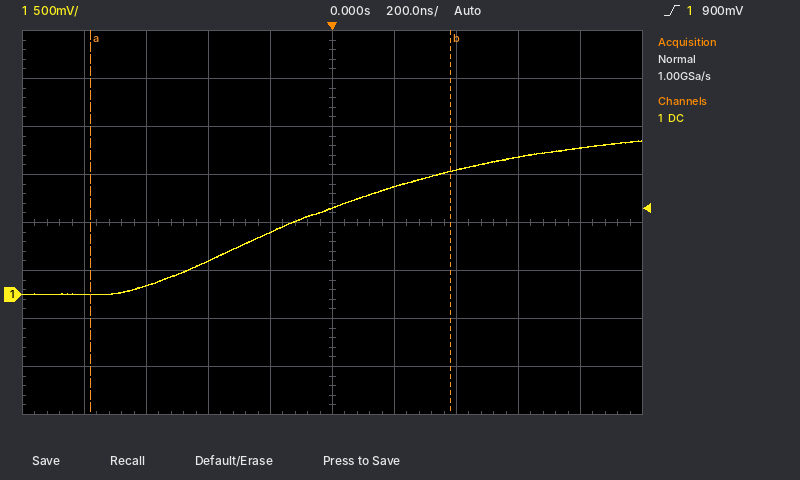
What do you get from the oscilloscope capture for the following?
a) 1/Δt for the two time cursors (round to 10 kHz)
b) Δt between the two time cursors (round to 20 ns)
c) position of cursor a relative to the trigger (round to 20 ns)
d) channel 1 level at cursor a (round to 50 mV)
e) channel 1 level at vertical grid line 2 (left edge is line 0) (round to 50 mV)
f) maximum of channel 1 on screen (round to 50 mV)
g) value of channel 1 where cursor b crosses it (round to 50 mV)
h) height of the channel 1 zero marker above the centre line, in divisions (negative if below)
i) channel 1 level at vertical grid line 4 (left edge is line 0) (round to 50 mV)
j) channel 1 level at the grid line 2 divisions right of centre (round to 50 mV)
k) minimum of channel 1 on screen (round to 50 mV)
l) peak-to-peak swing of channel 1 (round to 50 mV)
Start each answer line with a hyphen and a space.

- 860 kHz
- 1.16 µs
- -780 ns
- 0 mV
- 100 mV
- 1.60 V
- 1.30 V
- -1.5 div
- 650 mV
- 1.30 V
- 0 mV
- 1.60 V
